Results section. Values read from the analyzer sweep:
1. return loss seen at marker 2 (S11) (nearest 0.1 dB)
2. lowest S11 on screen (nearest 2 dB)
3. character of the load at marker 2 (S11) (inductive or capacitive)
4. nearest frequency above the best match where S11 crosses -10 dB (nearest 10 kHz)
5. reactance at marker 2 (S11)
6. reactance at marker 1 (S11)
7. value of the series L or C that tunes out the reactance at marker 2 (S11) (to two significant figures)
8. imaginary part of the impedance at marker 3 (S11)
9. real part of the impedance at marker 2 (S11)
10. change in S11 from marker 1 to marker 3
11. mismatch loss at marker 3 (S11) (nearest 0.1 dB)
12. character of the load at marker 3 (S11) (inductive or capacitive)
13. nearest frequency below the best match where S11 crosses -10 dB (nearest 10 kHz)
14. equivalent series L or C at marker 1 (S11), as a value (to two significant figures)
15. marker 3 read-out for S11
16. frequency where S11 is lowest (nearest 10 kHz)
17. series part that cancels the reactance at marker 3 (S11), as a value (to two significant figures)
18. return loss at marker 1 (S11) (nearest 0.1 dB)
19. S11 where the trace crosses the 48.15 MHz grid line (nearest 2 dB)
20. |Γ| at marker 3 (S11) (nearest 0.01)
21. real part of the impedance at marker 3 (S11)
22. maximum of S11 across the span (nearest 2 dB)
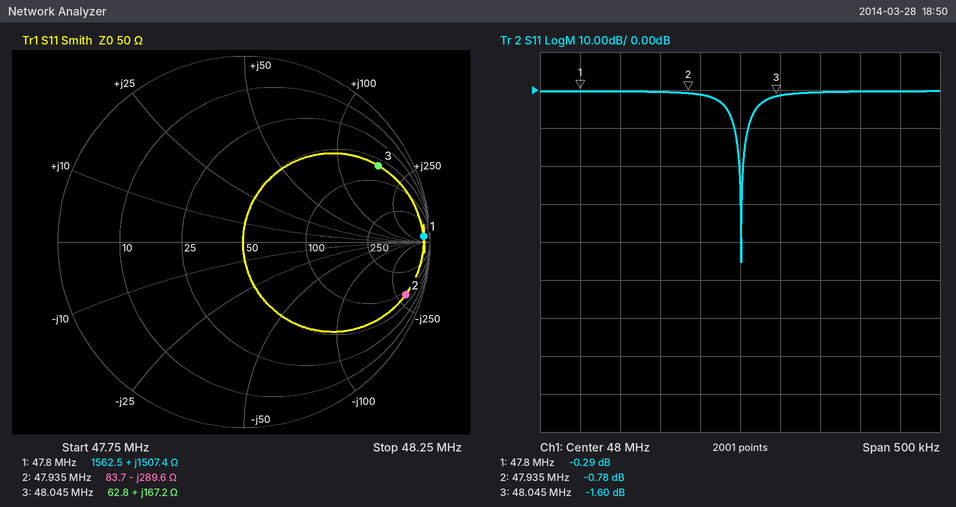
0.8 dB
-46 dB
capacitive
48.01 MHz
-289.6 Ω
+1507.4 Ω
960 nH
+167.2 Ω
83.7 Ω
-1.31 dB
5.1 dB
inductive
47.99 MHz
5.0 µH
-1.60 dB
48.00 MHz
20 pF
0.3 dB
0 dB
0.83
62.8 Ω
0 dB
